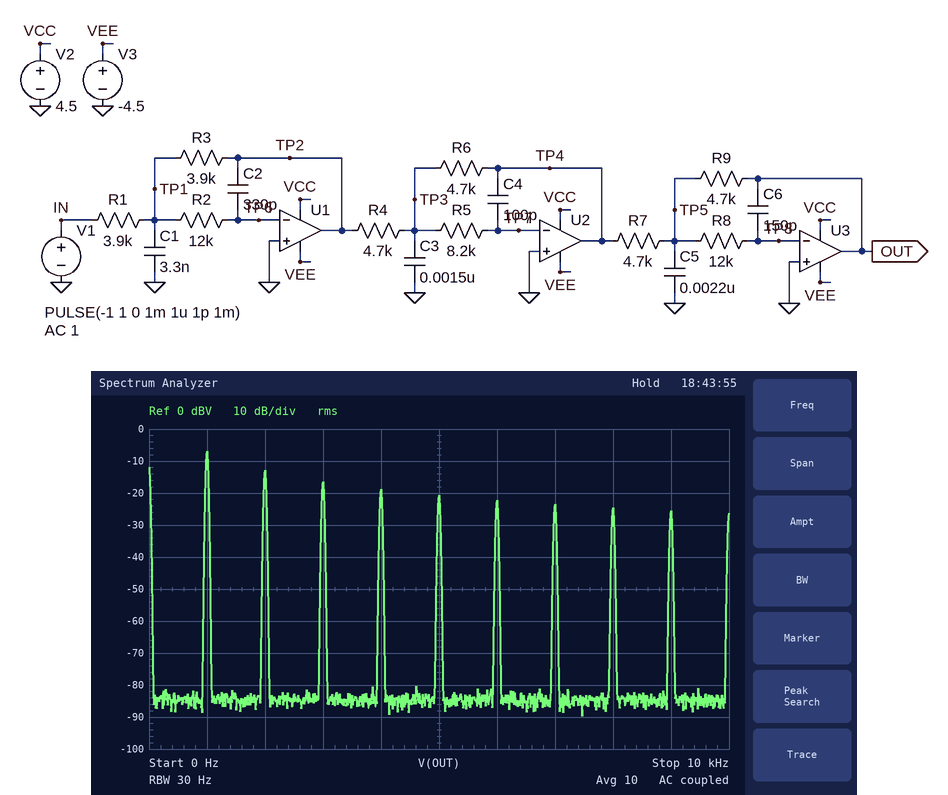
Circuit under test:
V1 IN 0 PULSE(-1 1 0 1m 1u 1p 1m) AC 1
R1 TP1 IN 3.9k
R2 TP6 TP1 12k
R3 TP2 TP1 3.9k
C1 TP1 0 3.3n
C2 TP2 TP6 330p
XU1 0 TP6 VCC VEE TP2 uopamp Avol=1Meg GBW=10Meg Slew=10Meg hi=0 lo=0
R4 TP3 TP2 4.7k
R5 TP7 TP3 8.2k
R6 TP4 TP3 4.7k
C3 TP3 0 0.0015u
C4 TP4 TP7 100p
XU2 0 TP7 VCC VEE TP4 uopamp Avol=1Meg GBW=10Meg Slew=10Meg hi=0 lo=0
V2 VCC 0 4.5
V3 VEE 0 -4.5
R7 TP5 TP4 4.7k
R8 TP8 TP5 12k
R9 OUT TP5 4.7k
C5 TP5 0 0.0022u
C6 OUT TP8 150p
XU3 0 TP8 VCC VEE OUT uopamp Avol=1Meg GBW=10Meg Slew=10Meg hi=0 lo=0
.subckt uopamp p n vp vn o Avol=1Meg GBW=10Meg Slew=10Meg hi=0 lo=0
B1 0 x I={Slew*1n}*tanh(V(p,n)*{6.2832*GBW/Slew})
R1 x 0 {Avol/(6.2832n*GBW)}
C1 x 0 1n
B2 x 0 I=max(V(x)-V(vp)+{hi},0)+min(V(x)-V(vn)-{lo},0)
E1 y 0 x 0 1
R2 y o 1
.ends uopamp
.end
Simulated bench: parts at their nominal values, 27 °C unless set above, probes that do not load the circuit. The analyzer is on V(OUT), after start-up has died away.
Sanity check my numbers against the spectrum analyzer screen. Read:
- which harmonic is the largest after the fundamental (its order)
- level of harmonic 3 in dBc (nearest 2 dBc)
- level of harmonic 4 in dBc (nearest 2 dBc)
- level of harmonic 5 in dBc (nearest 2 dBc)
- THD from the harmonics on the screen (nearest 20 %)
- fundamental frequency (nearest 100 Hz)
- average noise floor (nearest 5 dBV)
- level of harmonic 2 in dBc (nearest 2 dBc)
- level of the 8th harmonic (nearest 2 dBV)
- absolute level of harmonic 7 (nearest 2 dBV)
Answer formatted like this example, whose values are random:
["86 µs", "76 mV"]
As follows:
["2", "-10 dBc", "-12 dBc", "-14 dBc", "80 %", "1.0 kHz", "-85 dBV", "-6 dBc", "-24 dBV", "-24 dBV"]
